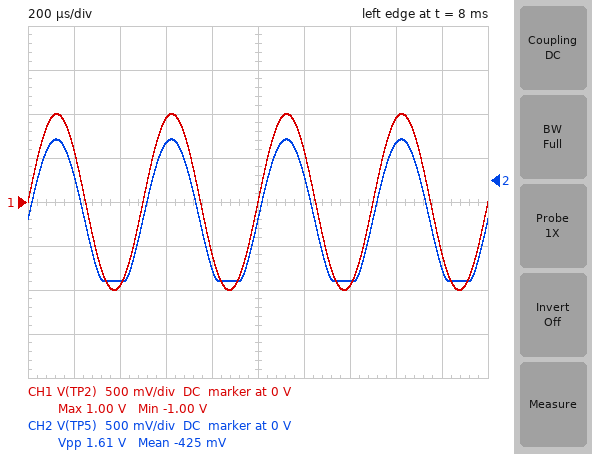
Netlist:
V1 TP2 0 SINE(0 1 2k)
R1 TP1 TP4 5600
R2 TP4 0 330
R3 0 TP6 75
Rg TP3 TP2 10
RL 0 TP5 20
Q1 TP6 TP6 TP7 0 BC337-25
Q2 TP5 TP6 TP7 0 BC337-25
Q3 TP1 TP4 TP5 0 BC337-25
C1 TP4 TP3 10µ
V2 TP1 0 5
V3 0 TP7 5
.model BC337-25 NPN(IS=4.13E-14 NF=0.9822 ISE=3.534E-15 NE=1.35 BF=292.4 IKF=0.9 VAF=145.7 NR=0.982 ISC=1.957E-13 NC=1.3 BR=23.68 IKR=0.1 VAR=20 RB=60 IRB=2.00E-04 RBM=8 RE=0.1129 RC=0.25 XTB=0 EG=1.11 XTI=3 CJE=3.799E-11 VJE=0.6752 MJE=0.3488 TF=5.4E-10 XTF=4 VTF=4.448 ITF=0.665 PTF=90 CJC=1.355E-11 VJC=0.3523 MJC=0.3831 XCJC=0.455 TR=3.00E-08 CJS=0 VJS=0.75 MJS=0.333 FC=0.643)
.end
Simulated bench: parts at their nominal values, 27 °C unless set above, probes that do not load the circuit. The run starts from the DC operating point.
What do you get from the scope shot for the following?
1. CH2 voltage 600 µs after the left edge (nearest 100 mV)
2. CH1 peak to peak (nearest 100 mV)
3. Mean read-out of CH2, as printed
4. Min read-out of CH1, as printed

400 mV
2.0 V
-425 mV
-1.00 V
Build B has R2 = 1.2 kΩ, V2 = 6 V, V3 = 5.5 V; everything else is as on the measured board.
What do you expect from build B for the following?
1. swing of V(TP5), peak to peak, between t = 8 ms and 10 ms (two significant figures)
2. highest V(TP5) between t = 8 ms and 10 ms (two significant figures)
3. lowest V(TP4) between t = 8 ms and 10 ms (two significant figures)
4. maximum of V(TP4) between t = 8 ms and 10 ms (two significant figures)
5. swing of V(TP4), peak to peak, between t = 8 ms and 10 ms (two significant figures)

1.9 V
1.0 V
-190 mV
1.8 V
2.0 V
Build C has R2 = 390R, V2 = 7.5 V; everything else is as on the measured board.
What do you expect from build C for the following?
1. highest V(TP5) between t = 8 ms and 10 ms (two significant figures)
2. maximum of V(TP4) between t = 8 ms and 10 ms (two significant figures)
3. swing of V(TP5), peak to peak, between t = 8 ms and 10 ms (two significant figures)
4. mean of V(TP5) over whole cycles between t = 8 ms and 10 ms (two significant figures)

650 mV
1.4 V
1.8 V
-270 mV
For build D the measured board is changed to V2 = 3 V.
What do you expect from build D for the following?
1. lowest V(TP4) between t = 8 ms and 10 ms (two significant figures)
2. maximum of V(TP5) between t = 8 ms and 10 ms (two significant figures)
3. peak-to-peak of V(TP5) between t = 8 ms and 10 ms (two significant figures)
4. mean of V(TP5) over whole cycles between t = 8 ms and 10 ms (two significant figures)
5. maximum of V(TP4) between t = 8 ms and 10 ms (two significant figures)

-840 mV
360 mV
1.5 V
-500 mV
1.1 V
